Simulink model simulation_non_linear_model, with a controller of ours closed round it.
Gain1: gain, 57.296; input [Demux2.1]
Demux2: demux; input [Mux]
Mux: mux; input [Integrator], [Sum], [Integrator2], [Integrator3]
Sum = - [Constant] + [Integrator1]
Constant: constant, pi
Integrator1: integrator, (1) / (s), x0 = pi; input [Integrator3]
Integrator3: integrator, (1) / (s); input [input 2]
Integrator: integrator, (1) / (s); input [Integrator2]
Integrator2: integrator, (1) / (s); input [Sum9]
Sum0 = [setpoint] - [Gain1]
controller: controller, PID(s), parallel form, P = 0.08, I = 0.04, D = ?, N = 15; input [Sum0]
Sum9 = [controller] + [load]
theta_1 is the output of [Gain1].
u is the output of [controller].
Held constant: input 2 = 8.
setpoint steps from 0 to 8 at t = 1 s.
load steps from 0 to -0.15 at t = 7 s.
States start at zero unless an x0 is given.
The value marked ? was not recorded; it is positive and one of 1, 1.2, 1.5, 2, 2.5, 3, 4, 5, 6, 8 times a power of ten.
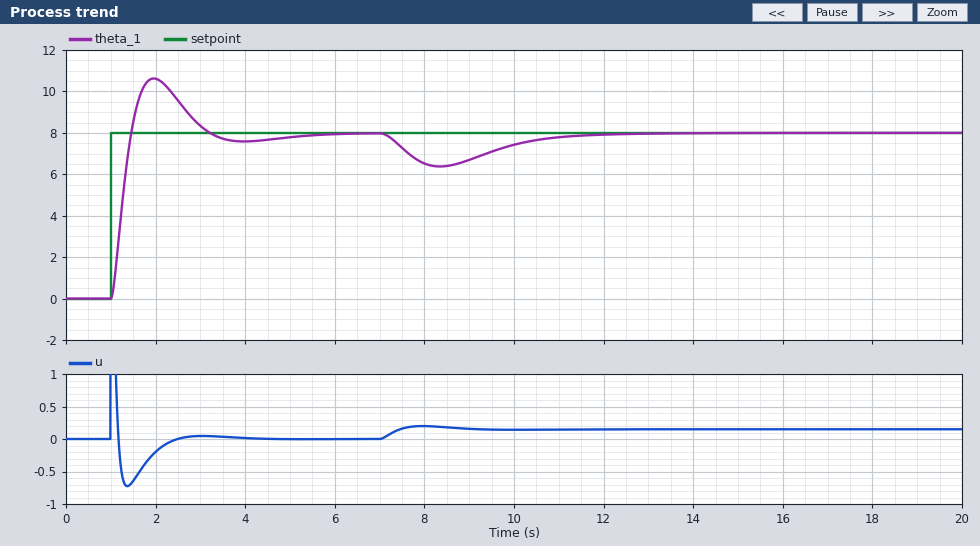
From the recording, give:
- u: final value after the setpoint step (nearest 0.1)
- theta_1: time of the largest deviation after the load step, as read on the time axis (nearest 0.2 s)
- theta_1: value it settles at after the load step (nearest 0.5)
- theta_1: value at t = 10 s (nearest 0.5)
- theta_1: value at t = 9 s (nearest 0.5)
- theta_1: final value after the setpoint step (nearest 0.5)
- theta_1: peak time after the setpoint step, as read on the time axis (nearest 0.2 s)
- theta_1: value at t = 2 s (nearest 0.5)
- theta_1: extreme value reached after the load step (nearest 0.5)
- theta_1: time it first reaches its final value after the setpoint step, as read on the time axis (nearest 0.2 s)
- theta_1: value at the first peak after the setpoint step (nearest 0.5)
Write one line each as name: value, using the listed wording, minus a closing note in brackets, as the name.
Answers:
u: final value after the setpoint step: 0.0
theta_1: time of the largest deviation after the load step, as read on the time axis: 8.4 s
theta_1: value it settles at after the load step: 8.0
theta_1: value at t = 10 s: 7.5
theta_1: value at t = 9 s: 6.5
theta_1: final value after the setpoint step: 8.0
theta_1: peak time after the setpoint step, as read on the time axis: 2.0 s
theta_1: value at t = 2 s: 10.5
theta_1: extreme value reached after the load step: 6.5
theta_1: time it first reaches its final value after the setpoint step, as read on the time axis: 1.4 s
theta_1: value at the first peak after the setpoint step: 10.5
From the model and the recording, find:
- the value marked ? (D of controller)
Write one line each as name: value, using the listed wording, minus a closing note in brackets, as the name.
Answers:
the value marked ?: 0.05
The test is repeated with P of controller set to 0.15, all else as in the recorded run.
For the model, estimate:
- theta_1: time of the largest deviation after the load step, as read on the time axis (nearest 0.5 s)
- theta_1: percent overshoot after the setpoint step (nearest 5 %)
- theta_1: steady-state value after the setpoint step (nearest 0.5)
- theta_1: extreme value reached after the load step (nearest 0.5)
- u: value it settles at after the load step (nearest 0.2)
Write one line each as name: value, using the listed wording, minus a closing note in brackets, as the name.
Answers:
theta_1: time of the largest deviation after the load step, as read on the time axis: 8.0 s
theta_1: percent overshoot after the setpoint step: 40 %
theta_1: steady-state value after the setpoint step: 8.0
theta_1: extreme value reached after the load step: 7.0
u: value it settles at after the load step: 0.2
